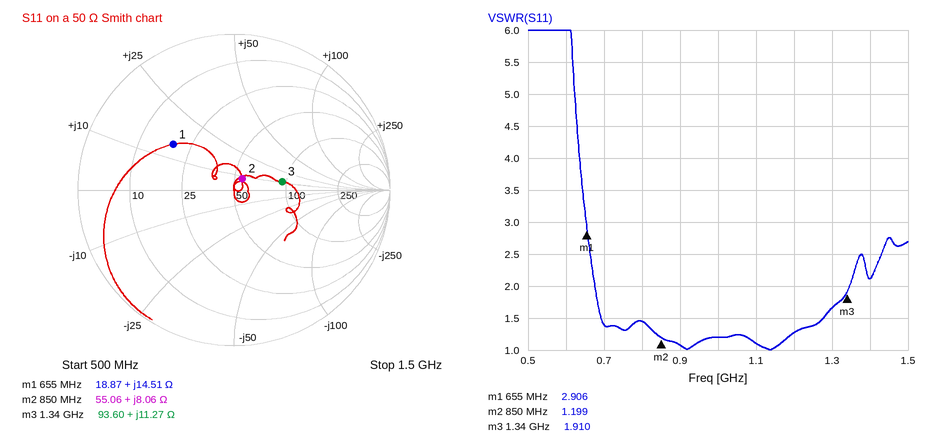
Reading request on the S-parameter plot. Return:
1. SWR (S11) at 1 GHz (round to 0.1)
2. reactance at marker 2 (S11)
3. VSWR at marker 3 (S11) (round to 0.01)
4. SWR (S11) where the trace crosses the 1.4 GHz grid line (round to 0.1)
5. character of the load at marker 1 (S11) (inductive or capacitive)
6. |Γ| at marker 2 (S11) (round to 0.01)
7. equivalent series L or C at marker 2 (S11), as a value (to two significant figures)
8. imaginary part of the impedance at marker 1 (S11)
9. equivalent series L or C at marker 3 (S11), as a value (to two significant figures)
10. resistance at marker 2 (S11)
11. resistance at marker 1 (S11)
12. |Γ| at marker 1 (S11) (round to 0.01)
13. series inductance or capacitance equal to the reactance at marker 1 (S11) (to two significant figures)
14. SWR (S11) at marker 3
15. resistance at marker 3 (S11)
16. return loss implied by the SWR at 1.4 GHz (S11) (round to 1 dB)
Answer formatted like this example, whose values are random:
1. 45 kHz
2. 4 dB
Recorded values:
1. 1.2
2. +8.06 Ω
3. 1.91
4. 2.1
5. inductive
6. 0.09
7. 1.5 nH
8. +14.51 Ω
9. 1.3 nH
10. 55.06 Ω
11. 18.87 Ω
12. 0.49
13. 3.5 nH
14. 1.910
15. 93.60 Ω
16. 9 dB
